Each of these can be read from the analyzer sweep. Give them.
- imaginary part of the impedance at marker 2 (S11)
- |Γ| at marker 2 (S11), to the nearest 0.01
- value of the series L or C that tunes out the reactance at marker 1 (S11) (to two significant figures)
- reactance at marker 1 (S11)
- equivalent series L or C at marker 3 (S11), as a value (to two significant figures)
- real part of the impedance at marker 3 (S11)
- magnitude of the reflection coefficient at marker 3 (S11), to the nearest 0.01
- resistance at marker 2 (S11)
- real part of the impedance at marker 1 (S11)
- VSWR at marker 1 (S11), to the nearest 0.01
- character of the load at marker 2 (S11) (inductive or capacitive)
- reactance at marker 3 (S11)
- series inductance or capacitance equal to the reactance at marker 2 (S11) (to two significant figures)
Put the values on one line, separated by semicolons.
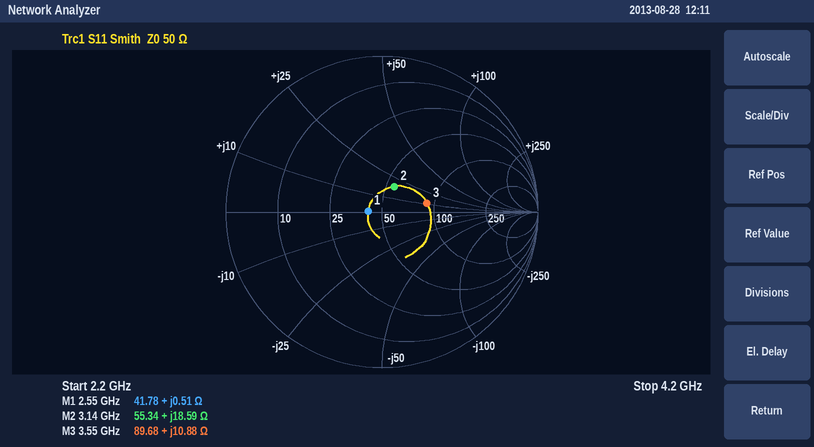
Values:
+18.59 Ω; 0.18; 120 pF; +0.51 Ω; 490 pH; 89.68 Ω; 0.29; 55.34 Ω; 41.78 Ω; 1.20; inductive; +10.88 Ω; 940 pH
